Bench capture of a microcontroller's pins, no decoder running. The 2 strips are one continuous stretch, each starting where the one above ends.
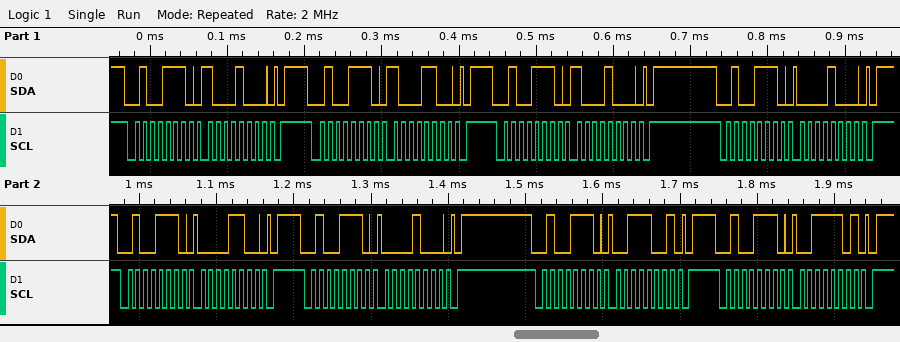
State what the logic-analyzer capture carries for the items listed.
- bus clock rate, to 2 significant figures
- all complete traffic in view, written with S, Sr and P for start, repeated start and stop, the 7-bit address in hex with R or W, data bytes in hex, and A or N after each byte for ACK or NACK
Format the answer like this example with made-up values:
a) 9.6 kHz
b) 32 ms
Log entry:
a) 100 kHz
b) S 27W A 88 A P S 27W A 8C A P S 27W A 88 A P S 27W A 08 A P S 27W A 0C A P S 27W A 08 A P S 27W A 39 A P S 27W A 3D A P
